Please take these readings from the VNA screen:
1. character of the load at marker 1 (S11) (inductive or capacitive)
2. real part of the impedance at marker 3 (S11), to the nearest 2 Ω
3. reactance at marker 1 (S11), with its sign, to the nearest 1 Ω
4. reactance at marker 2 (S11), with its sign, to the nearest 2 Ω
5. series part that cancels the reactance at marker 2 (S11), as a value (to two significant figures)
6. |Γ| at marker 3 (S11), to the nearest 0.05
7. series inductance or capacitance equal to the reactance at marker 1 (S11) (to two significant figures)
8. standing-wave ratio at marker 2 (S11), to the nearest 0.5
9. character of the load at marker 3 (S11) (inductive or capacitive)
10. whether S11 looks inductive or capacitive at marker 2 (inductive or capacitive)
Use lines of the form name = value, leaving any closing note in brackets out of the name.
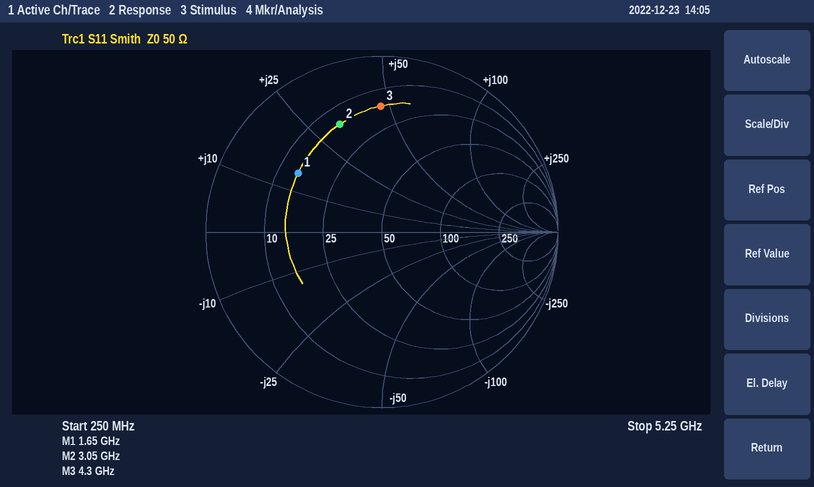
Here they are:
character of the load at marker 1 (S11) = inductive
real part of the impedance at marker 3 (S11), to the nearest 2 Ω = 16 Ω
reactance at marker 1 (S11), with its sign, to the nearest 1 Ω = +15 Ω
reactance at marker 2 (S11), with its sign, to the nearest 2 Ω = +32 Ω
series part that cancels the reactance at marker 2 (S11), as a value = 1.6 pF
|Γ| at marker 3 (S11), to the nearest 0.05 = 0.70
series inductance or capacitance equal to the reactance at marker 1 (S11) = 1.4 nH
standing-wave ratio at marker 2 (S11), to the nearest 0.5 = 5.0
character of the load at marker 3 (S11) = inductive
whether S11 looks inductive or capacitive at marker 2 = inductive
